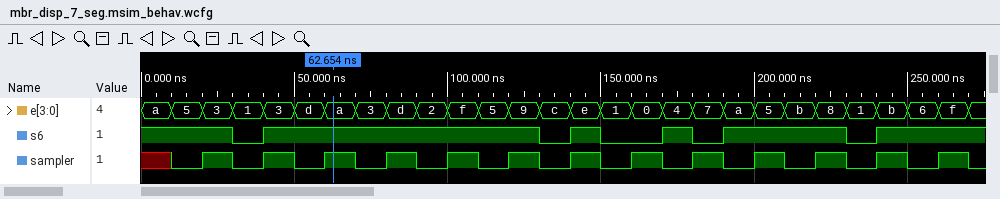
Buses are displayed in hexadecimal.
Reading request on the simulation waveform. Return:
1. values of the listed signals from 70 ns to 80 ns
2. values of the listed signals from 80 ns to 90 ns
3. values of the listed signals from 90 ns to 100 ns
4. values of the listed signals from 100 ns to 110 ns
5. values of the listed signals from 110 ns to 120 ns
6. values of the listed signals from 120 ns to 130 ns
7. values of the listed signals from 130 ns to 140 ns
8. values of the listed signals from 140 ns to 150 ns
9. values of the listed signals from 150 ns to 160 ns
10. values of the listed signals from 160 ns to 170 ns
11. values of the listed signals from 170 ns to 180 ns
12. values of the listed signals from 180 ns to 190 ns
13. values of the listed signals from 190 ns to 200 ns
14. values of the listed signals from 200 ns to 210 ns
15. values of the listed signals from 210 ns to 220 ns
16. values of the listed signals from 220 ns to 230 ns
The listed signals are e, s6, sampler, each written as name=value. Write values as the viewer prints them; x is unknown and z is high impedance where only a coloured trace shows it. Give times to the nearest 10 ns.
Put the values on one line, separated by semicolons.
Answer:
e=3, s6=1, sampler=0; e=d, s6=1, sampler=1; e=2, s6=1, sampler=0; e=f, s6=1, sampler=1; e=5, s6=1, sampler=0; e=9, s6=1, sampler=1; e=c, s6=0, sampler=0; e=e, s6=1, sampler=1; e=1, s6=0, sampler=0; e=0, s6=0, sampler=1; e=4, s6=1, sampler=0; e=7, s6=0, sampler=1; e=a, s6=1, sampler=0; e=5, s6=1, sampler=1; e=b, s6=1, sampler=0; e=8, s6=1, sampler=1
